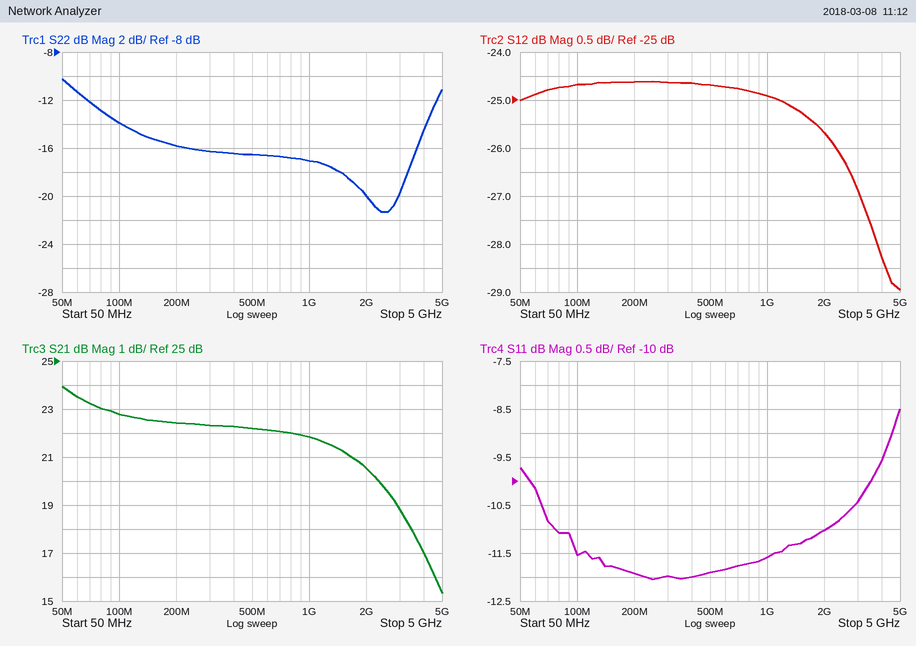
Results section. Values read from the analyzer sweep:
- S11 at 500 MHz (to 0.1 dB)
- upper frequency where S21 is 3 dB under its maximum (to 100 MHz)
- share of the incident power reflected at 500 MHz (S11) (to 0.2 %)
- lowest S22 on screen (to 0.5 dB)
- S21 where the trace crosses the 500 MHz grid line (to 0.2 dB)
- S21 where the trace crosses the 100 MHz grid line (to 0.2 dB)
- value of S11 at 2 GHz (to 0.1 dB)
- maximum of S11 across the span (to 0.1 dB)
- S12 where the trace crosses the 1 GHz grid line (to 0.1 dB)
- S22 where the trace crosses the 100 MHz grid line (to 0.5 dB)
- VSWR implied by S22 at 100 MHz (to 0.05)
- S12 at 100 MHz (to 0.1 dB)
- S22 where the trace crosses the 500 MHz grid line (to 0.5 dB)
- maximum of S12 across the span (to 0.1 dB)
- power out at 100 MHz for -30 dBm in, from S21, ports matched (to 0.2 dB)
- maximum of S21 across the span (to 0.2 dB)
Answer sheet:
-11.9 dB
1.7 GHz
6.4 %
-21.5 dB
22.2 dB
22.8 dB
-11.0 dB
-8.5 dB
-24.9 dB
-14.0 dB
1.50
-24.7 dB
-16.5 dB
-24.6 dB
-7.2 dBm
24.0 dB
